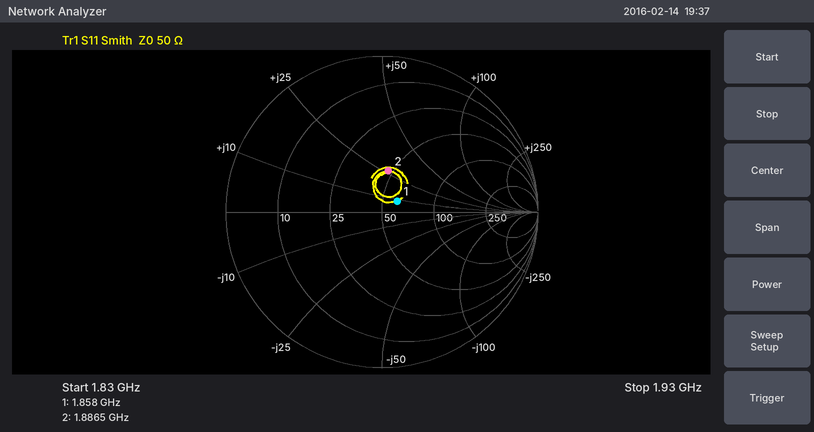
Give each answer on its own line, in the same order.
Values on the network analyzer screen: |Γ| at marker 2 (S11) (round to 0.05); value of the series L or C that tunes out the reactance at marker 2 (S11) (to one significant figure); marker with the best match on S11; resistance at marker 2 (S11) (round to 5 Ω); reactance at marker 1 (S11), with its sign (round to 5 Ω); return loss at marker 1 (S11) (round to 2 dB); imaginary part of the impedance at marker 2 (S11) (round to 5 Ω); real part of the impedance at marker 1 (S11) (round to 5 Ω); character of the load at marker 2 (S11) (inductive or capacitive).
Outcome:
0.25
3 pF
marker 1
45 Ω
+10 Ω
18 dB
+25 Ω
60 Ω
inductive
